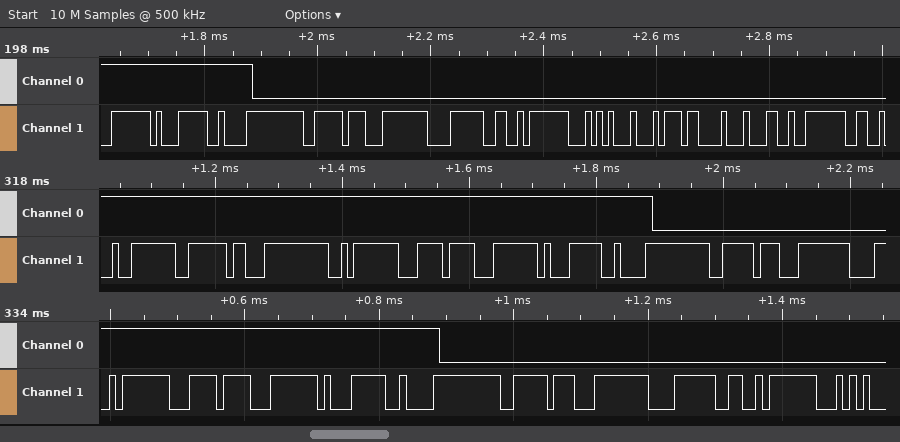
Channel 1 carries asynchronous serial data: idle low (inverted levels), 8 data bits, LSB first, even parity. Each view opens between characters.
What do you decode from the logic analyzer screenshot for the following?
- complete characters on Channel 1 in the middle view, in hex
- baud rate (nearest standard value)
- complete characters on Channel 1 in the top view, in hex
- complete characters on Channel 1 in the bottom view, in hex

03, 20, 00, 01, 08, 40, B0, 00, 10, 80
100000 baud
40, B0, 00, 10, 80, 60, 01, 75, 91, 77, 03
01, 08, 40, B0, 00, 10, 80, 60, 01
